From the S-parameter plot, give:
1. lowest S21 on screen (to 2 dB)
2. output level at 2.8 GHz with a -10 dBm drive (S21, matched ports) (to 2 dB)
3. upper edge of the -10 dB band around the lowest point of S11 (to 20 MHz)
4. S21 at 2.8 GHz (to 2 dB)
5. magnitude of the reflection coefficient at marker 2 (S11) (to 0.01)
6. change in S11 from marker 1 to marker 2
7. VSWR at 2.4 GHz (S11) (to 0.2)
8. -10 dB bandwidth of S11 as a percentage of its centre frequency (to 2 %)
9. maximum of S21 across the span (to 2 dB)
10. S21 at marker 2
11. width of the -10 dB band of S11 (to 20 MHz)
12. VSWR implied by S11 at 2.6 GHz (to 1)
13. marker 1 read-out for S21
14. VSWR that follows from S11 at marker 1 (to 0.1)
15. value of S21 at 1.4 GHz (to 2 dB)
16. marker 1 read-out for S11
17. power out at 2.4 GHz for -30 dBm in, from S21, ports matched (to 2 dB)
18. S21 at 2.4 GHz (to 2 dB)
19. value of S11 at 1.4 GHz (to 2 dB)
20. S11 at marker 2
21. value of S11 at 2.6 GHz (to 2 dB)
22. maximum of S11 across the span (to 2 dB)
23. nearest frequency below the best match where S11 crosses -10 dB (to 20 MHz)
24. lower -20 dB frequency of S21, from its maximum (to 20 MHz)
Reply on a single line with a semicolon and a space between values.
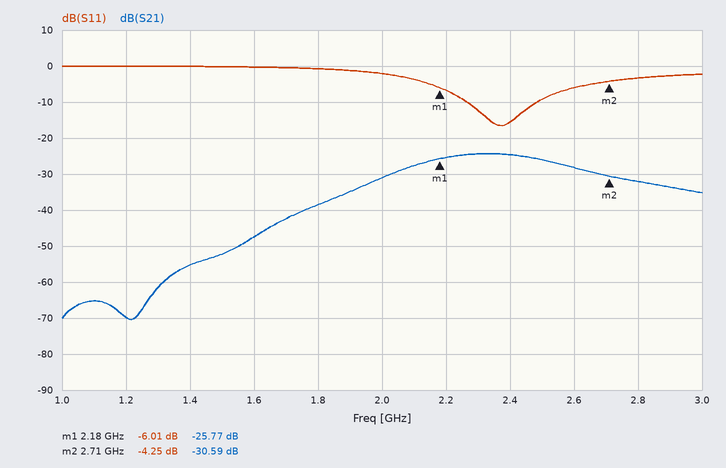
-70 dB; -42 dBm; 2.48 GHz; -32 dB; 0.61; 1.76 dB; 1.4; 10 %; -24 dB; -30.59 dB; 220 MHz; 3; -25.77 dB; 3.0; -56 dB; -6.01 dB; -54 dBm; -24 dB; 0 dB; -4.25 dB; -6 dB; 0 dB; 2.26 GHz; 1.66 GHz
